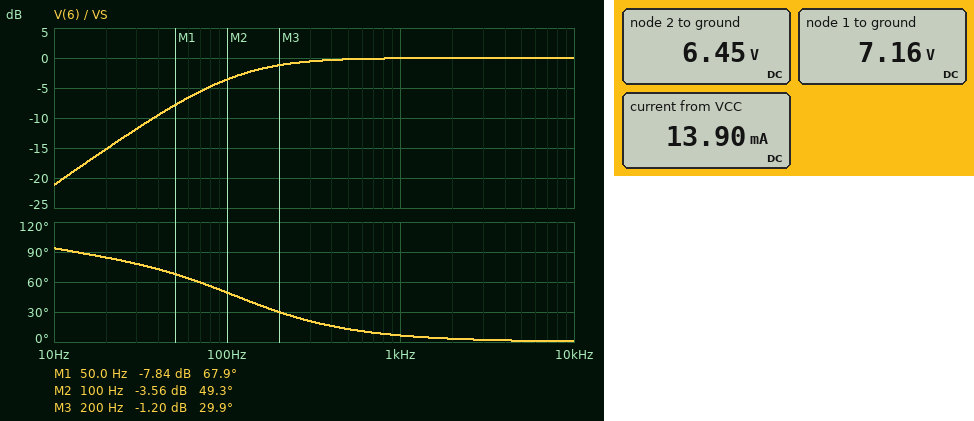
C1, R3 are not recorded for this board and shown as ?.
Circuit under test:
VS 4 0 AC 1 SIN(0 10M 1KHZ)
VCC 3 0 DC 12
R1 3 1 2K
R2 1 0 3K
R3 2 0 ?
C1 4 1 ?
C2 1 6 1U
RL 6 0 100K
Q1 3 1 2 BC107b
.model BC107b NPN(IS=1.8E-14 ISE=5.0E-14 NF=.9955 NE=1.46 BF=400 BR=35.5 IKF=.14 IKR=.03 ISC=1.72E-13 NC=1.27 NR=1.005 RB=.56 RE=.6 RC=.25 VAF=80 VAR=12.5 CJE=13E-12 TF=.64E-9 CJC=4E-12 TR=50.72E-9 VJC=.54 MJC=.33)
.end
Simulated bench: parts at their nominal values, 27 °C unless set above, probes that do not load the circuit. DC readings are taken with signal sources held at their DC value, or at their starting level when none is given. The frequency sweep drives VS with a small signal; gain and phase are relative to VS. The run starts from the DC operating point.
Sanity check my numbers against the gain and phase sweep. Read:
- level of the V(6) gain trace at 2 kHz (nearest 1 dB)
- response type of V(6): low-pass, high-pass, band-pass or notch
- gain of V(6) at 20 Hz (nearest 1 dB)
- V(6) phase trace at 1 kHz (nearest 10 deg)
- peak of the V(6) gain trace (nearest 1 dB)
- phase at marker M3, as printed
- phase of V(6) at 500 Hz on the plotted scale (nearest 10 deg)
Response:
0 dB
high-pass
-15 dB
10 deg
0 dB
29.9 deg
10 deg
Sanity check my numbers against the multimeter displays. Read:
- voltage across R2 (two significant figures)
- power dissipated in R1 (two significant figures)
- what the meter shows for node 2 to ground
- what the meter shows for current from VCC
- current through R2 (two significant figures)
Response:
7.2 V
12 mW
6.45 V
13.90 mA
2.4 mA
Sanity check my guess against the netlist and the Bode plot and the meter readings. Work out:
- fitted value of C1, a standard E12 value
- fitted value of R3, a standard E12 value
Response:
1.2 µF
560 Ω
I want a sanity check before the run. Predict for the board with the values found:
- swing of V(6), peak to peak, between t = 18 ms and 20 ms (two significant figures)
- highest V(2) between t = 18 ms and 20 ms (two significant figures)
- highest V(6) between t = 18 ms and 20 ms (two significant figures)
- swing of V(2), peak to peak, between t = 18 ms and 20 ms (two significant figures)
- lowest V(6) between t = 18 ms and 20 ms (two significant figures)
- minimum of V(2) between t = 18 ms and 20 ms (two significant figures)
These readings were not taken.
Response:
20 mV
6.5 V
9.9 mV
20 mV
-9.9 mV
6.4 V
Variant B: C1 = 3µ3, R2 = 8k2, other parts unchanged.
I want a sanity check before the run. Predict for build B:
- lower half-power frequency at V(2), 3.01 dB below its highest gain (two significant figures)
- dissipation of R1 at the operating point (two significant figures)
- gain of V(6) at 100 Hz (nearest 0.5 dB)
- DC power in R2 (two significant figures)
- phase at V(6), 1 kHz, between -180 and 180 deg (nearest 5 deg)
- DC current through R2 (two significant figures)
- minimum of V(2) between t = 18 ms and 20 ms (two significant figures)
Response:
31 Hz
3.0 mW
-0.5 dB
11 mW
0 deg
1.2 mA
8.8 V
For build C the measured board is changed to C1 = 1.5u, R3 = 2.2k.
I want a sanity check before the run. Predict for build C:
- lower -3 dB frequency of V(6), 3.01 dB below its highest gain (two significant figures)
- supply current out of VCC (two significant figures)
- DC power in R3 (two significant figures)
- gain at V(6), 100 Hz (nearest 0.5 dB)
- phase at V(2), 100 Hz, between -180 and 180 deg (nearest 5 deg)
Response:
90 Hz
5.4 mA
19 mW
-2.5 dB
40 deg
